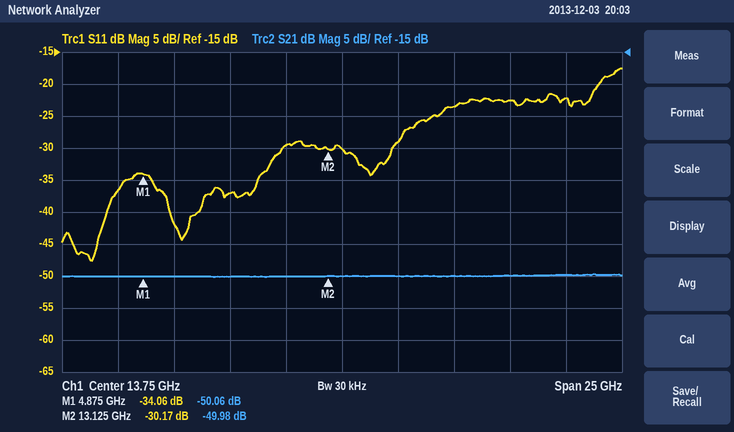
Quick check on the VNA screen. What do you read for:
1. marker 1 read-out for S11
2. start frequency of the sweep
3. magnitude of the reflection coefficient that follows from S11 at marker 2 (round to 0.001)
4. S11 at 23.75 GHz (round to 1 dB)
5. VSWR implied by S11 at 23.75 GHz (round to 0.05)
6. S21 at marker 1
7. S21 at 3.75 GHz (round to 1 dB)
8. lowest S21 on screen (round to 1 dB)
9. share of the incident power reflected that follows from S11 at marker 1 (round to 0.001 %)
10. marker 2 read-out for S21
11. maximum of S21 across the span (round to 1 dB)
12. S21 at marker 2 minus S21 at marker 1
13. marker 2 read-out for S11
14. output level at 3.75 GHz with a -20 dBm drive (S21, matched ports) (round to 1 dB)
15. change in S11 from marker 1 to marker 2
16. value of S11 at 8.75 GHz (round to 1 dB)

-34.06 dB
1.25 GHz
0.031
-22 dB
1.15
-50.06 dB
-50 dB
-50 dB
0.039 %
-49.98 dB
-50 dB
0.08 dB
-30.17 dB
-70 dBm
3.89 dB
-37 dB
